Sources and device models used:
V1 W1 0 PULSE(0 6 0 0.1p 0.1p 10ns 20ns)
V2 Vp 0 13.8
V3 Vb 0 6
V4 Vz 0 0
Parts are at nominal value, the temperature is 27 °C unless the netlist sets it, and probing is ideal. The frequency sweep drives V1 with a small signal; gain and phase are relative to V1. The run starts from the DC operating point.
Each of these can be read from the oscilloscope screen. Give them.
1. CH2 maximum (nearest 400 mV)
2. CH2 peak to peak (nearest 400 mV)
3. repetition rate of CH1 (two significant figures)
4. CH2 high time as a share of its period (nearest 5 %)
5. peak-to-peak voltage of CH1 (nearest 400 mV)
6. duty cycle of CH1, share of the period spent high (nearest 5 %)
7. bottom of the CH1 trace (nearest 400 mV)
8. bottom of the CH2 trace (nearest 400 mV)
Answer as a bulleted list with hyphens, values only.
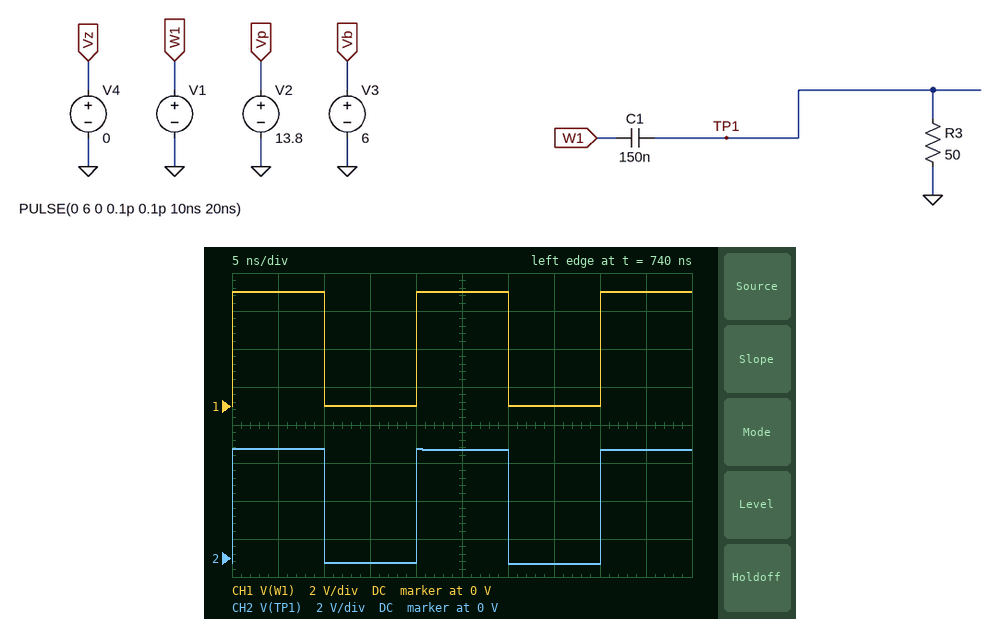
- 5.6 V
- 6.0 V
- 50 MHz
- 50 %
- 6.0 V
- 50 %
- 0 V
- -400 mV
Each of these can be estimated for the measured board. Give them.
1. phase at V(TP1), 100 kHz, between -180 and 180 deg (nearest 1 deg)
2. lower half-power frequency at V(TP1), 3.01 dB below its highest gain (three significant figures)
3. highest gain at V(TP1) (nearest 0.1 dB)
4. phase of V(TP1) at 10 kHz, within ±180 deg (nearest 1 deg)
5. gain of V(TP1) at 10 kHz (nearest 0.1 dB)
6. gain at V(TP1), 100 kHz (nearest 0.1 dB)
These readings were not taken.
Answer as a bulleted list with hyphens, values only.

- 12 deg
- 21.2 kHz
- 0 dB
- 65 deg
- -7.4 dB
- -0.2 dB
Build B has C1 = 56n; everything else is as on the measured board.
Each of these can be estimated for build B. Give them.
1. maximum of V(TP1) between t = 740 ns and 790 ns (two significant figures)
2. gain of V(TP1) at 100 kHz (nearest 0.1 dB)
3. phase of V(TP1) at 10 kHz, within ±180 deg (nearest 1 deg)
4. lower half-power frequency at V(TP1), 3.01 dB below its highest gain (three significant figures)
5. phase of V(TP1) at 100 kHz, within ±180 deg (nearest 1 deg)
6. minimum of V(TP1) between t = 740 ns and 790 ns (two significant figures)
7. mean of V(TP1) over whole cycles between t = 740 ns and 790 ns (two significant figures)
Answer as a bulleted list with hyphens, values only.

- 5.3 V
- -1.2 dB
- 80 deg
- 56.8 kHz
- 30 deg
- -750 mV
- 2.3 V
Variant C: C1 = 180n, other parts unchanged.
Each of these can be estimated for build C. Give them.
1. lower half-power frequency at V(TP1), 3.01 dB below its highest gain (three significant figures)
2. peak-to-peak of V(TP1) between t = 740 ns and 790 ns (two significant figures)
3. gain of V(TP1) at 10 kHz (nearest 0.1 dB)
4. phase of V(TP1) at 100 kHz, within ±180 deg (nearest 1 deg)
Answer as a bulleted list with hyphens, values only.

- 17.7 kHz
- 6.0 V
- -6.2 dB
- 10 deg
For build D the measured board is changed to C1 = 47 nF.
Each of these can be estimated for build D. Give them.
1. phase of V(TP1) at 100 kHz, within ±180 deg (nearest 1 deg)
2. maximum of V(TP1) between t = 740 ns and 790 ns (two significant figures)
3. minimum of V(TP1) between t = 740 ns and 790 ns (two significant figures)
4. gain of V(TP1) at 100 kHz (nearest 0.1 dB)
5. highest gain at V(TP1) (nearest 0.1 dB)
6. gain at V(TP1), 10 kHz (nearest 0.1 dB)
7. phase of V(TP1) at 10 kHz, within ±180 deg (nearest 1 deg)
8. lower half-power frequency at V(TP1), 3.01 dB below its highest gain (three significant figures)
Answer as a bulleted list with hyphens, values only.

- 34 deg
- 5.2 V
- -870 mV
- -1.6 dB
- 0 dB
- -16.7 dB
- 82 deg
- 67.7 kHz
